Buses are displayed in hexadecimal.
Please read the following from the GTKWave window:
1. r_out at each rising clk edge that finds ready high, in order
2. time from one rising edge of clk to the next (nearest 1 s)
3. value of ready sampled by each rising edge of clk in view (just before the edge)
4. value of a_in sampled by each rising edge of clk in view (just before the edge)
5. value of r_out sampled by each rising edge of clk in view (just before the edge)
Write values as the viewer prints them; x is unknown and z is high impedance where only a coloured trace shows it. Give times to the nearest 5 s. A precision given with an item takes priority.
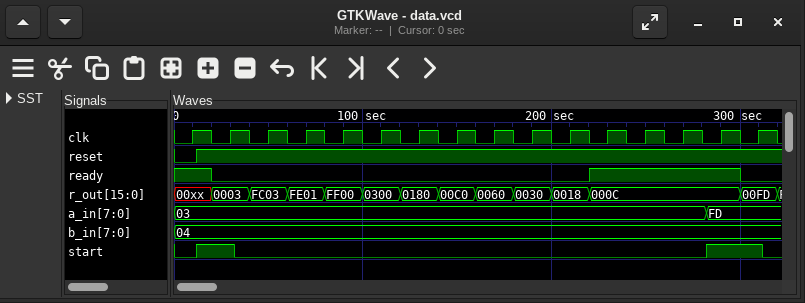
00xx, 000C, 000C, 000C, 000C
20 s
1 0 0 0 0 0 0 0 0 0 0 1 1 1 1 0
03, 03, 03, 03, 03, 03, 03, 03, 03, 03, 03, 03, 03, 03, FD, FD
00xx, 0003, FC03, FE01, FF00, 0300, 0180, 00C0, 0060, 0030, 0018, 000C, 000C, 000C, 000C, 00FD
